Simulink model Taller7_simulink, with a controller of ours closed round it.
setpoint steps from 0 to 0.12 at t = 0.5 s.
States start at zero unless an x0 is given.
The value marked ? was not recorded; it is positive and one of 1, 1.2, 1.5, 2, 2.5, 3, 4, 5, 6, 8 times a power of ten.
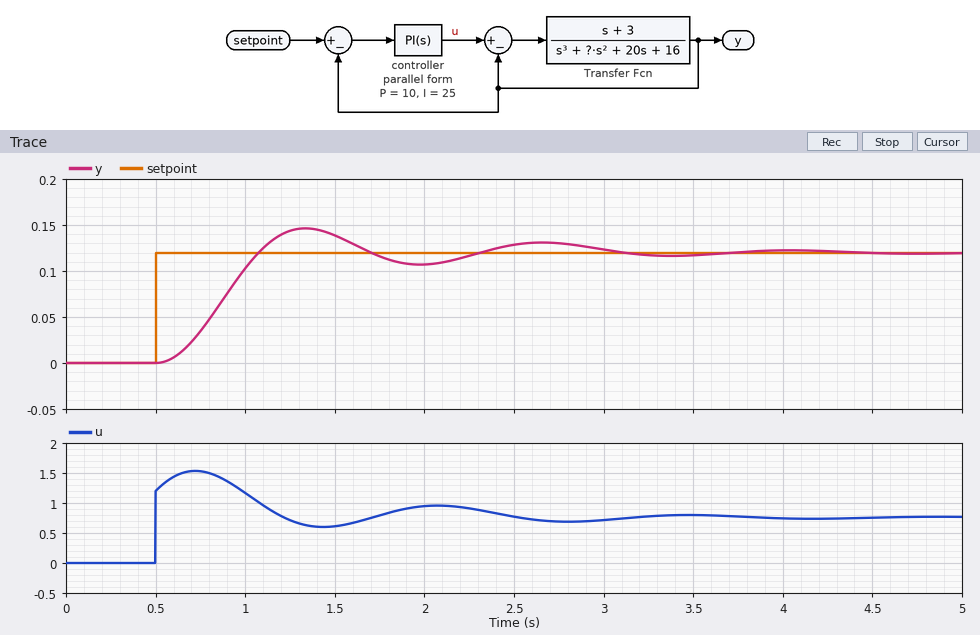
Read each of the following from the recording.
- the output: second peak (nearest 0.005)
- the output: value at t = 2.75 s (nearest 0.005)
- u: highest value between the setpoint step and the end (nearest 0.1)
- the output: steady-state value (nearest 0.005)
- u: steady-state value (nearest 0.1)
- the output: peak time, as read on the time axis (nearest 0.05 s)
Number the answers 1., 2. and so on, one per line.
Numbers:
1. 0.130
2. 0.130
3. 1.5
4. 0.120
5. 0.8
6. 1.35 s
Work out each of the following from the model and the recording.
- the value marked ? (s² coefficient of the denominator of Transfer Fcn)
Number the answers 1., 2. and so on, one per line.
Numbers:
1. 5
